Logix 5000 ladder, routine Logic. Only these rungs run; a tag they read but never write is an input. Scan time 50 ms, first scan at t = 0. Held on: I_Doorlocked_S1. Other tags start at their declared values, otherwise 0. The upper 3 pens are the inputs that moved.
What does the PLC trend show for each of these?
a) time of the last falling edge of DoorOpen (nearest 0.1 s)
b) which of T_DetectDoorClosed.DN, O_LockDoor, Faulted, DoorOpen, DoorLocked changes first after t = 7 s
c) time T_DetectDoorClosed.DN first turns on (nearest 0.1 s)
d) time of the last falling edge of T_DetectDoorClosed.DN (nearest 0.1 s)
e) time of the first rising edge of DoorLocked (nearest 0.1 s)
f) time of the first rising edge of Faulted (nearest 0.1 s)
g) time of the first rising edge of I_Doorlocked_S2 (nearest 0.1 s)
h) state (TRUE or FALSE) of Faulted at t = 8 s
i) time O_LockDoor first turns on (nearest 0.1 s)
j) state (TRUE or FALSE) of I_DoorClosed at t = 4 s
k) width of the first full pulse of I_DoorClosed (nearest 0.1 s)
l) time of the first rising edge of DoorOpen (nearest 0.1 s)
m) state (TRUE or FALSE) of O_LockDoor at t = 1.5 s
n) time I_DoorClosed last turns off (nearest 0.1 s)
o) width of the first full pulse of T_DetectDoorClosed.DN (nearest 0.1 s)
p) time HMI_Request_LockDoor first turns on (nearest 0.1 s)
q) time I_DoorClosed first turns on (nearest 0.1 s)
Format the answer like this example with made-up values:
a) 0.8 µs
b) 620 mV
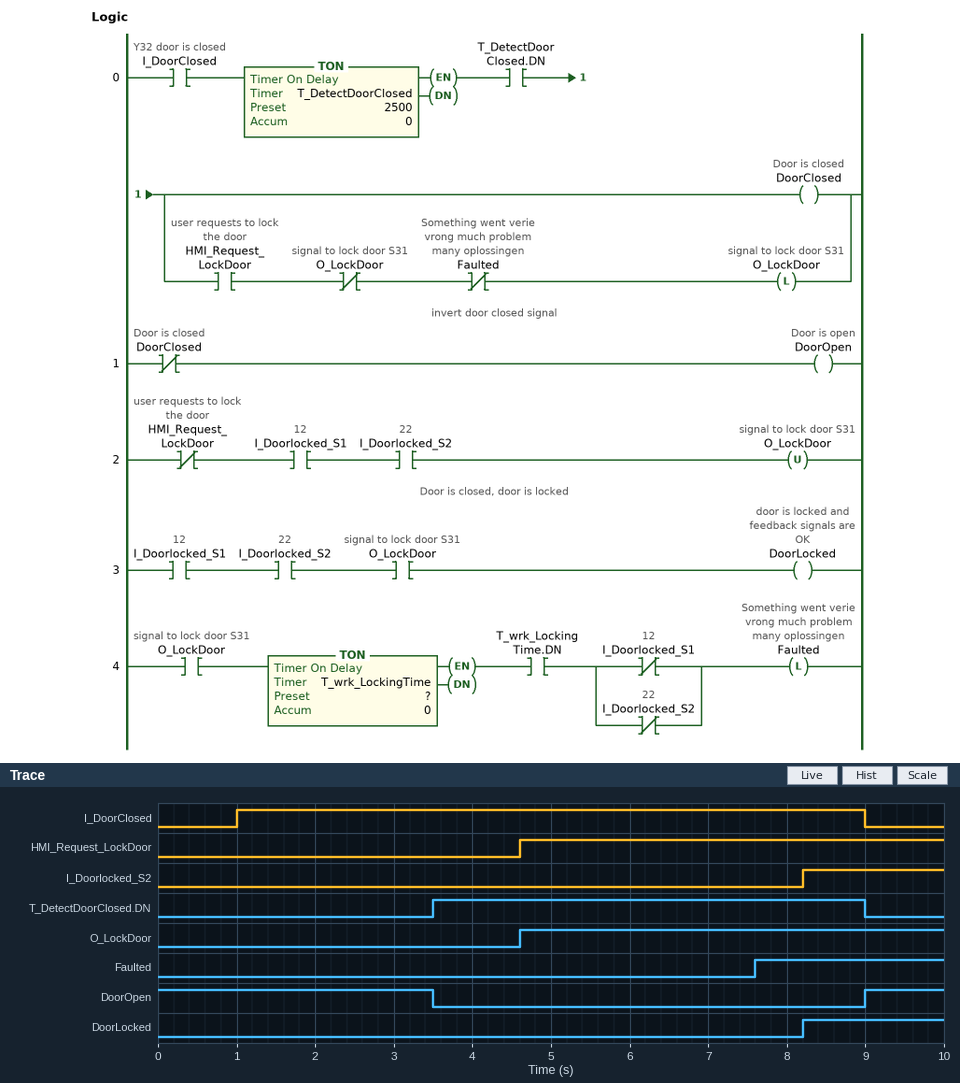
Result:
a) 3.5 s
b) Faulted
c) 3.5 s
d) 9.0 s
e) 8.2 s
f) 7.6 s
g) 8.2 s
h) TRUE
i) 4.6 s
j) TRUE
k) 8.0 s
l) 9.0 s
m) FALSE
n) 9.0 s
o) 5.5 s
p) 4.6 s
q) 1.0 s
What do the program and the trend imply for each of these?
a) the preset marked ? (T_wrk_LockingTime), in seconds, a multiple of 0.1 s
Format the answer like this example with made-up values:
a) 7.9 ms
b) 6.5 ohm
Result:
a) 3.0 s
